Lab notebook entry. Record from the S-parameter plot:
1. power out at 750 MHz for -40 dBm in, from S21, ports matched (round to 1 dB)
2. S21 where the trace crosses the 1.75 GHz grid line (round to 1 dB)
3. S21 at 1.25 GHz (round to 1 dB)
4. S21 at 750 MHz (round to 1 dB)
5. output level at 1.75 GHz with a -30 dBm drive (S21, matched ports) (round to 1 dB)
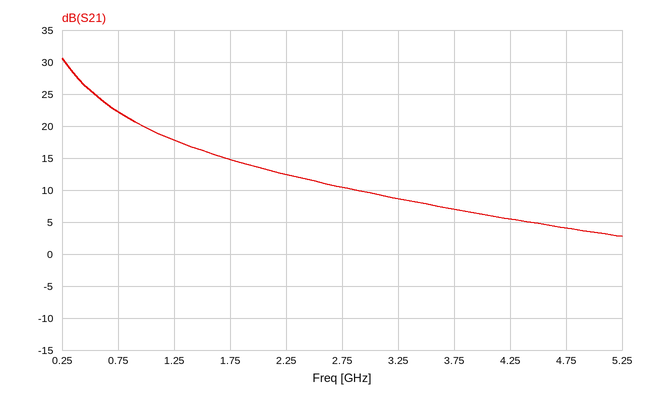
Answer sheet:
-18 dBm
15 dB
18 dB
22 dB
-15 dBm
